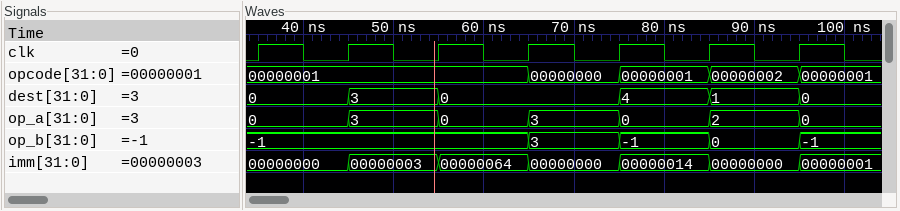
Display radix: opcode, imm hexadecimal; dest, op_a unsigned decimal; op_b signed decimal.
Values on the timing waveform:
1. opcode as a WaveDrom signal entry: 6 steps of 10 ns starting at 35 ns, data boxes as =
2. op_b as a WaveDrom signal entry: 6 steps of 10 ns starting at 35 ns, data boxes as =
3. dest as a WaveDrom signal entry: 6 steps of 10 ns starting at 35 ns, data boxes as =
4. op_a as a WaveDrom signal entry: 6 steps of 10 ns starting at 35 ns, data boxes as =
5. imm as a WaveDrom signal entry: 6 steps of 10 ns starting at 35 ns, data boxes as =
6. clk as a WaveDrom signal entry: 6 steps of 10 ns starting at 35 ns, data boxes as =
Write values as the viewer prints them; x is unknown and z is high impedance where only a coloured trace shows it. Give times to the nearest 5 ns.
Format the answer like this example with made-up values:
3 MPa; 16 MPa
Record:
{name: 'opcode', wave: '=..===', data: '00000001 00000000 00000001 00000002'}; {name: 'op_b', wave: '=..===', data: '-1 3 -1 0'}; {name: 'dest', wave: '===.==', data: '0 3 0 4 1'}; {name: 'op_a', wave: '======', data: '0 3 0 3 0 2'}; {name: 'imm', wave: '======', data: '00000000 00000003 00000064 00000000 00000014 00000000'}; {name: 'clk', wave: 'p.....'}
